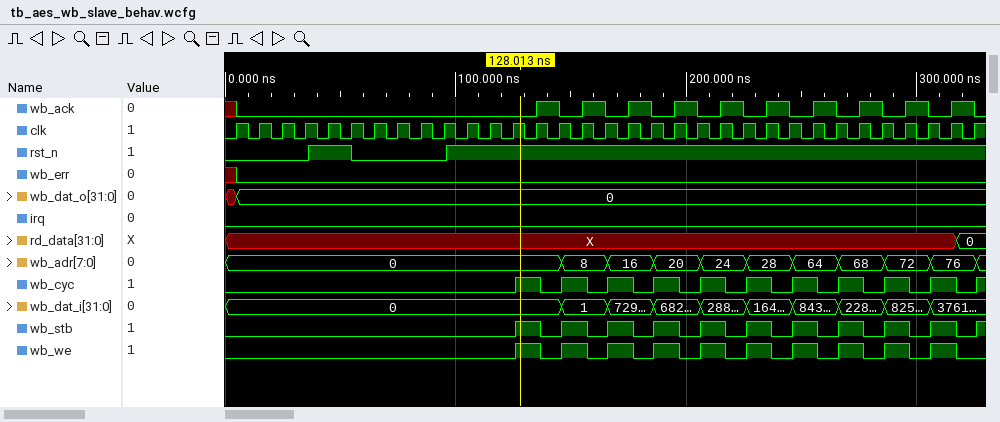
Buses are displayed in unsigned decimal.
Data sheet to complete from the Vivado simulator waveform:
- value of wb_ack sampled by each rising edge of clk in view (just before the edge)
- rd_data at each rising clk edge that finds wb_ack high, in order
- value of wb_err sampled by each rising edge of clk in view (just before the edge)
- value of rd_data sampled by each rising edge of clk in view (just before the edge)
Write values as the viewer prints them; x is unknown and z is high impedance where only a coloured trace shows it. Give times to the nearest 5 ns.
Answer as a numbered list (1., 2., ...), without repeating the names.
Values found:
1. x 0 0 0 0 0 0 0 0 0 0 0 0 0 1 0 1 0 1 0 1 0 1 0 1 0 1 0 1 0 1 0 1
2. X, X, X, X, X, X, X, X, X, 0
3. x 0 0 0 0 0 0 0 0 0 0 0 0 0 0 0 0 0 0 0 0 0 0 0 0 0 0 0 0 0 0 0 0
4. X, X, X, X, X, X, X, X, X, X, X, X, X, X, X, X, X, X, X, X, X, X, X, X, X, X, X, X, X, X, X, X, 0
